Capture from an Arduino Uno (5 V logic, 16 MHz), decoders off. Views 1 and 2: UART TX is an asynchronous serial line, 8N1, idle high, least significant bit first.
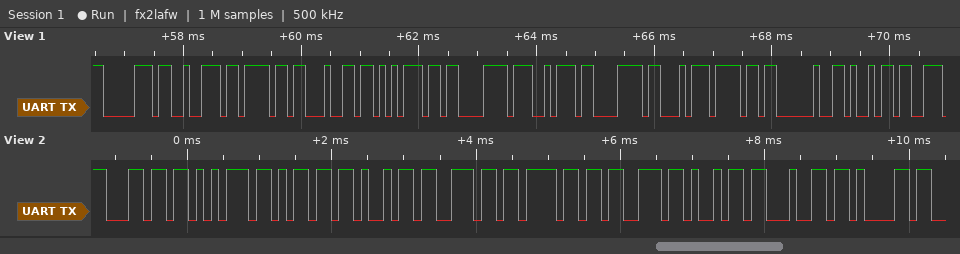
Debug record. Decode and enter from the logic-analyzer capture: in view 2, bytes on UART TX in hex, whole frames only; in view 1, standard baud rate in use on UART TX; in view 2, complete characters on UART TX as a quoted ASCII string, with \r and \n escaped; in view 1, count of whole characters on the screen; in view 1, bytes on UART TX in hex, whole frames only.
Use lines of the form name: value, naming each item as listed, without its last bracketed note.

in view 2, bytes on UART TX in hex, whole frames only: 6C 75 6D 69 6E 6F 73 69 64 61
in view 1, standard baud rate in use on UART TX: 9600 baud
in view 2, complete characters on UART TX as a quoted ASCII string, with \r and \n escaped: "luminosida"
in view 1, count of whole characters on the screen: 12
in view 1, bytes on UART TX in hex, whole frames only: 70 72 6F 64 75 C3 A7 C3 A3 6F 20 69
